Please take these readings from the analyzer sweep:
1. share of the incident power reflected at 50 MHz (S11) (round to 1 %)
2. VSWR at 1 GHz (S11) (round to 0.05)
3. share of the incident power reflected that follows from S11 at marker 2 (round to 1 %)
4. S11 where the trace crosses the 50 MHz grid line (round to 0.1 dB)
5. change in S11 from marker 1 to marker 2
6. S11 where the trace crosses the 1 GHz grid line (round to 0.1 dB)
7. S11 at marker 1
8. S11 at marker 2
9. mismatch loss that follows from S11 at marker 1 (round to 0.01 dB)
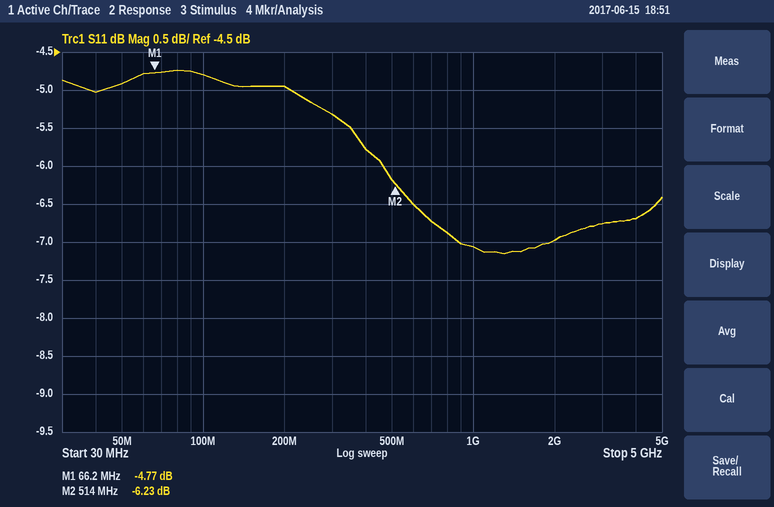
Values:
32 %
2.60
24 %
-4.9 dB
-1.46 dB
-7.1 dB
-4.77 dB
-6.23 dB
1.76 dB
